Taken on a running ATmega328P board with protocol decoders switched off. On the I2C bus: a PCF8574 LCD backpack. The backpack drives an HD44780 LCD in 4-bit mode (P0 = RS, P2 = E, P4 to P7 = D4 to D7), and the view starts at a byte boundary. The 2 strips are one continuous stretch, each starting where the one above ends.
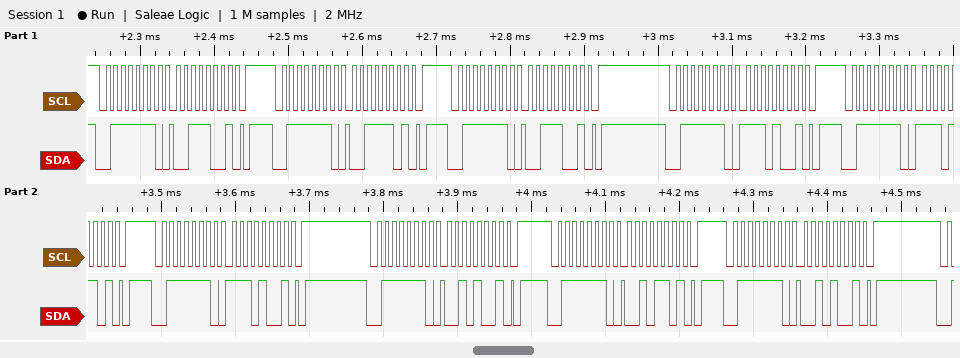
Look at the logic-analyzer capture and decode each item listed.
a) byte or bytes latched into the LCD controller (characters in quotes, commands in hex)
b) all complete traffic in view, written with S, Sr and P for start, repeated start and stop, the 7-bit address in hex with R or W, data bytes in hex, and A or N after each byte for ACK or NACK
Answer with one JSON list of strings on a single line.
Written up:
["'>'", "S 3FW A 39 A P S 3FW A 3D A P S 3FW A 39 A P S 3FW A E9 A P S 3FW A ED A P S 3FW A E9 A P S 3FW A 29 A P S 3FW A 2D A P S 3FW A 29 A P"]
